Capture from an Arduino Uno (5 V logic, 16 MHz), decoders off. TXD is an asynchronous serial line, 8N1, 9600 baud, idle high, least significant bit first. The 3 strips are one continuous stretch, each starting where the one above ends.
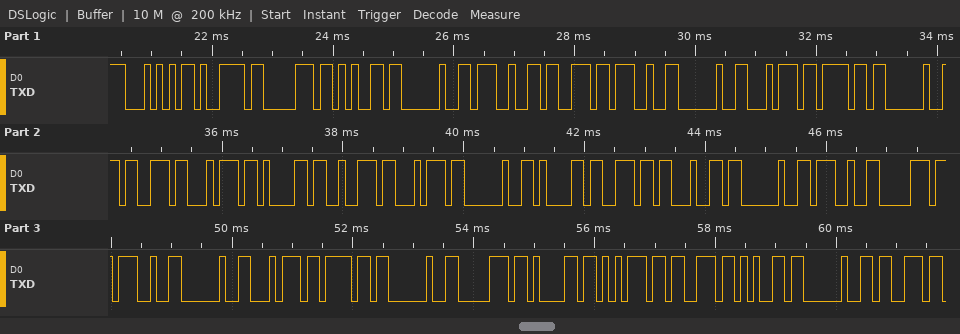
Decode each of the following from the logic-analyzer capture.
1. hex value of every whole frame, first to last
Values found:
0x54 0x79 0x70 0x65 0x20 0x27 0x73 0x27 0x20 0x74 0x6F 0x20 0x73 0x74 0x61 0x72 0x74 0x20 0x61 0x6E 0x64 0x20 0x27 0x70 0x27 0x20 0x74 0x6F 0x20 0x70 0x61 0x75 0x73 0x65 0x20 0x73
